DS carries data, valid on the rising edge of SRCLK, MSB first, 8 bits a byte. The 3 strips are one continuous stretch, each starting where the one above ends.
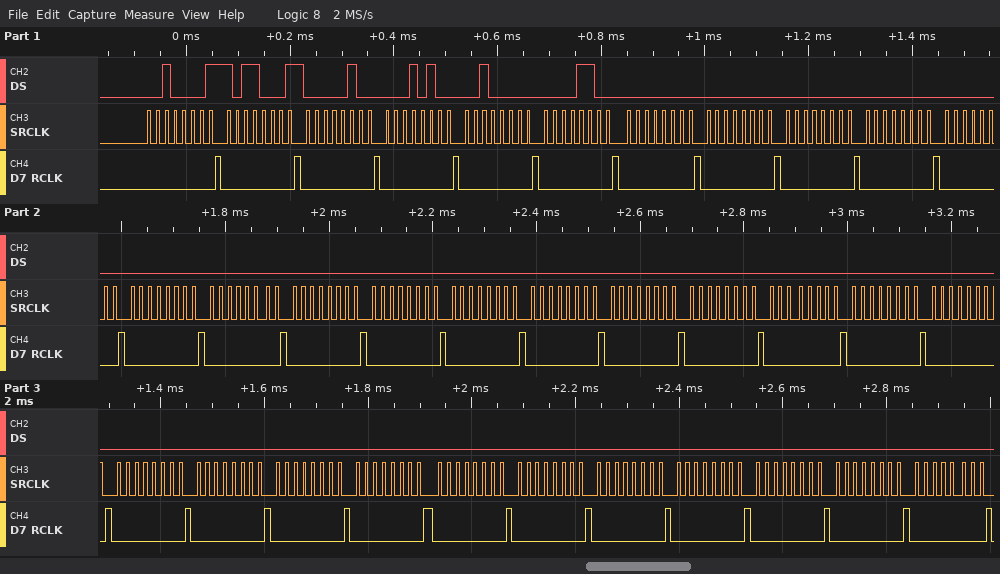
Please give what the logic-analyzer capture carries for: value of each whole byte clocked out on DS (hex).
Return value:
0x21 0xB1 0x04 0x14 0x20 0x0C 0x00 0x00 0x00 0x00 0x00 0x00 0x00 0x00 0x00 0x00 0x00 0x00 0x00 0x00 0x00 0x00 0x00 0x00 0x00 0x00 0x00 0x00 0x00 0x00 0x00 0x00 0x00
